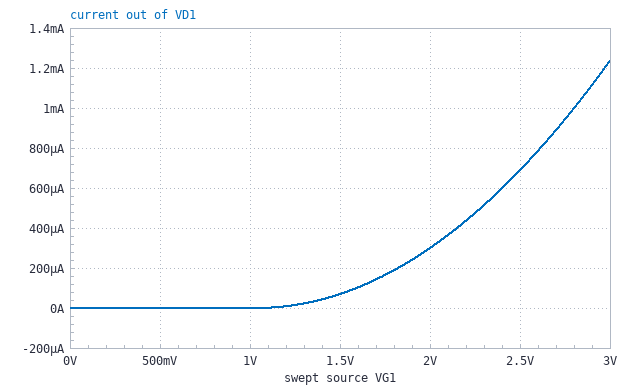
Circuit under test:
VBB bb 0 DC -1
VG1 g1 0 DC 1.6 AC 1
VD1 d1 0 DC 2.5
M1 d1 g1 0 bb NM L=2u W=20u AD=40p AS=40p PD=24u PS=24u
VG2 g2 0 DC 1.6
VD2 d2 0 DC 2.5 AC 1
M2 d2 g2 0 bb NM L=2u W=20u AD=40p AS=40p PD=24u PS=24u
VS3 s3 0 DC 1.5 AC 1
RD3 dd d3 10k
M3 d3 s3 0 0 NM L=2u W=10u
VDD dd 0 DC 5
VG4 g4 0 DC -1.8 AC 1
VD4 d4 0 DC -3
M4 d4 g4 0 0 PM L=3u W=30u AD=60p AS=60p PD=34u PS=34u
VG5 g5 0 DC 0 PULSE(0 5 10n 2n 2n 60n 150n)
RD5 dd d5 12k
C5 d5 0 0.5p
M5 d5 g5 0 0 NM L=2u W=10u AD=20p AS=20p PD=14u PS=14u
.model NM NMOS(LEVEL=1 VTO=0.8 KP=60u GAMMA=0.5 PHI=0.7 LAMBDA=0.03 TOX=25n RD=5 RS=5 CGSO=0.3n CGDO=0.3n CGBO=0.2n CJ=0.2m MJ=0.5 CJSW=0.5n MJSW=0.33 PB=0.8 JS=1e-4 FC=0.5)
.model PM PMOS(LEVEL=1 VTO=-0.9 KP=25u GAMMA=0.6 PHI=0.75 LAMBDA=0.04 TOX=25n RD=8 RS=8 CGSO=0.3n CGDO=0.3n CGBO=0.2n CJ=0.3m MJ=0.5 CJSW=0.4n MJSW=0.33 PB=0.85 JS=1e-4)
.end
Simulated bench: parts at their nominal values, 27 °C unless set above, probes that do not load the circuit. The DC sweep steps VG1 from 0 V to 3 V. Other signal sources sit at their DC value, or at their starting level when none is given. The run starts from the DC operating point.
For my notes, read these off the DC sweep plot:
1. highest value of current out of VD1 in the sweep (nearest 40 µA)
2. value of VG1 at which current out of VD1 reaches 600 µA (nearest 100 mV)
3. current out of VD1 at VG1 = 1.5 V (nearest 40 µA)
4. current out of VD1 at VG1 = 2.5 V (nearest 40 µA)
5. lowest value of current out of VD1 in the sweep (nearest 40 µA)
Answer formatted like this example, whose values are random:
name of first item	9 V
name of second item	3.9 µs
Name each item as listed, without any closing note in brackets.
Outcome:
highest value of current out of VD1 in the sweep	1.24 mA
value of VG1 at which current out of VD1 reaches 600 µA	2.4 V
current out of VD1 at VG1 = 1.5 V	80 µA
current out of VD1 at VG1 = 2.5 V	680 µA
lowest value of current out of VD1 in the sweep	0 A
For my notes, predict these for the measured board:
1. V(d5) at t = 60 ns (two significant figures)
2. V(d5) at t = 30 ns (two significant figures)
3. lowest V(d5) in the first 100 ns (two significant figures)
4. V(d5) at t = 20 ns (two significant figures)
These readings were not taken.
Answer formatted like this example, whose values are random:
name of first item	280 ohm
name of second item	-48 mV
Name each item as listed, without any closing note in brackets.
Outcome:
V(d5) at t = 60 ns	320 mV
V(d5) at t = 30 ns	320 mV
lowest V(d5) in the first 100 ns	320 mV
V(d5) at t = 20 ns	320 mV
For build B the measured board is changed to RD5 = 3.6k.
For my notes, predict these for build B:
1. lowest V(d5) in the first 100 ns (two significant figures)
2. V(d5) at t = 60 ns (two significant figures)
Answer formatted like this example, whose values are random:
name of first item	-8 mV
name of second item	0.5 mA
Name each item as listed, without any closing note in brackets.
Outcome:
lowest V(d5) in the first 100 ns	980 mV
V(d5) at t = 60 ns	990 mV
